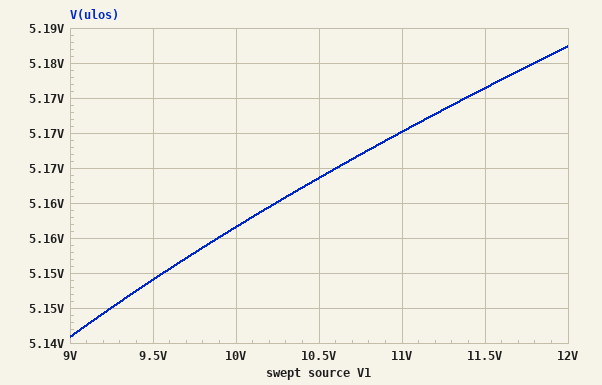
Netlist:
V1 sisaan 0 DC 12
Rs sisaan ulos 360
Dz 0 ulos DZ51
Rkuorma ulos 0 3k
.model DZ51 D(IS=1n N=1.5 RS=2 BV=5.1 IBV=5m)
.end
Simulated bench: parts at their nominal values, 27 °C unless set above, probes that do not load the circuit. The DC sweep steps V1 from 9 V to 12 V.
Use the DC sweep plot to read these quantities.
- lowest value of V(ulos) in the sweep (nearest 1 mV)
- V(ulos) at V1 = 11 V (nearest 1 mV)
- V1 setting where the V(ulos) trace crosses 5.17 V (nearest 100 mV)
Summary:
5.141 V
5.170 V
11.0 V
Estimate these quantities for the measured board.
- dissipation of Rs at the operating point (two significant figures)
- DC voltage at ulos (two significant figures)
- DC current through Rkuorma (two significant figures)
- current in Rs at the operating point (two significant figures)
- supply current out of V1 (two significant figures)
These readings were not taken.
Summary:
130 mW
5.2 V
1.7 mA
19 mA
19 mA
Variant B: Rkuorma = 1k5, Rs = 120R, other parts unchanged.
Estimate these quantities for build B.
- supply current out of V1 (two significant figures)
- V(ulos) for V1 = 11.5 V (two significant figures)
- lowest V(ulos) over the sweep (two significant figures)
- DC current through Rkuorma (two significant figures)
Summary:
56 mA
5.3 V
5.2 V
3.5 mA
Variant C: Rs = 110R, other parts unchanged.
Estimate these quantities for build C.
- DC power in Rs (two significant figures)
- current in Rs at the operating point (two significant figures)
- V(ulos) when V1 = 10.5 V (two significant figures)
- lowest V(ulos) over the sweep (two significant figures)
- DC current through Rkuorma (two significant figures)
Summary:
410 mW
61 mA
5.3 V
5.2 V
1.8 mA
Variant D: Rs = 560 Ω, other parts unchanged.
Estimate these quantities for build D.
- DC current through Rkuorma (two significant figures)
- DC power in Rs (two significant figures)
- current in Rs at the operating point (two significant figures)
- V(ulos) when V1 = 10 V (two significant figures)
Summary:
1.7 mA
84 mW
12 mA
5.1 V
